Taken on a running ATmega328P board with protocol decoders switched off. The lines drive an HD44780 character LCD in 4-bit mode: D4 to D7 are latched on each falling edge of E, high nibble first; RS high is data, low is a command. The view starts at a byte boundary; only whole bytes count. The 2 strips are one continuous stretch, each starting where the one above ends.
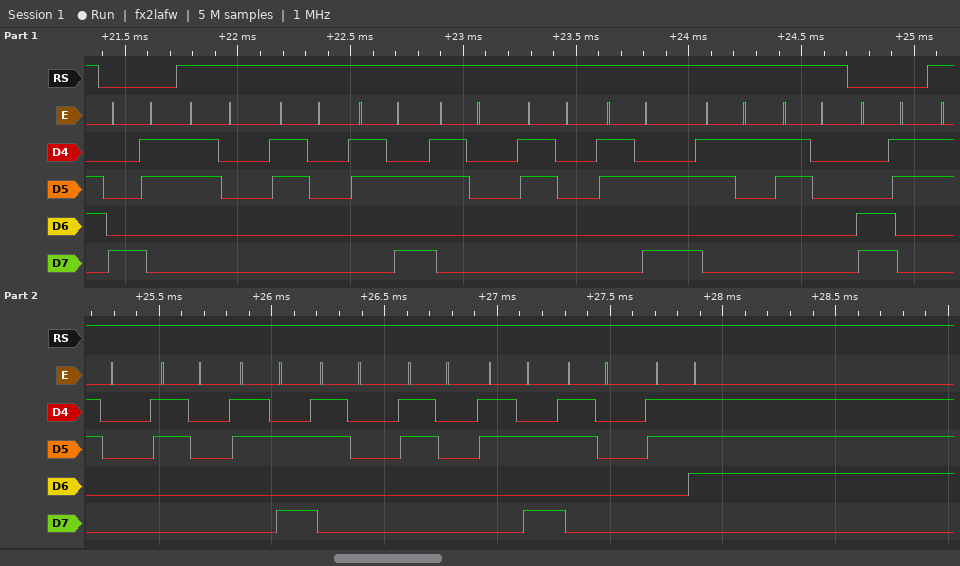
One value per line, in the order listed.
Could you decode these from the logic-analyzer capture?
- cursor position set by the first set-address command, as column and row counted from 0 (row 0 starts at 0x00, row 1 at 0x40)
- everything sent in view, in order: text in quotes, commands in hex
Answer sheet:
column 3, row 0
0x83 "00:00:10" 0xC3 "00:00:07"
